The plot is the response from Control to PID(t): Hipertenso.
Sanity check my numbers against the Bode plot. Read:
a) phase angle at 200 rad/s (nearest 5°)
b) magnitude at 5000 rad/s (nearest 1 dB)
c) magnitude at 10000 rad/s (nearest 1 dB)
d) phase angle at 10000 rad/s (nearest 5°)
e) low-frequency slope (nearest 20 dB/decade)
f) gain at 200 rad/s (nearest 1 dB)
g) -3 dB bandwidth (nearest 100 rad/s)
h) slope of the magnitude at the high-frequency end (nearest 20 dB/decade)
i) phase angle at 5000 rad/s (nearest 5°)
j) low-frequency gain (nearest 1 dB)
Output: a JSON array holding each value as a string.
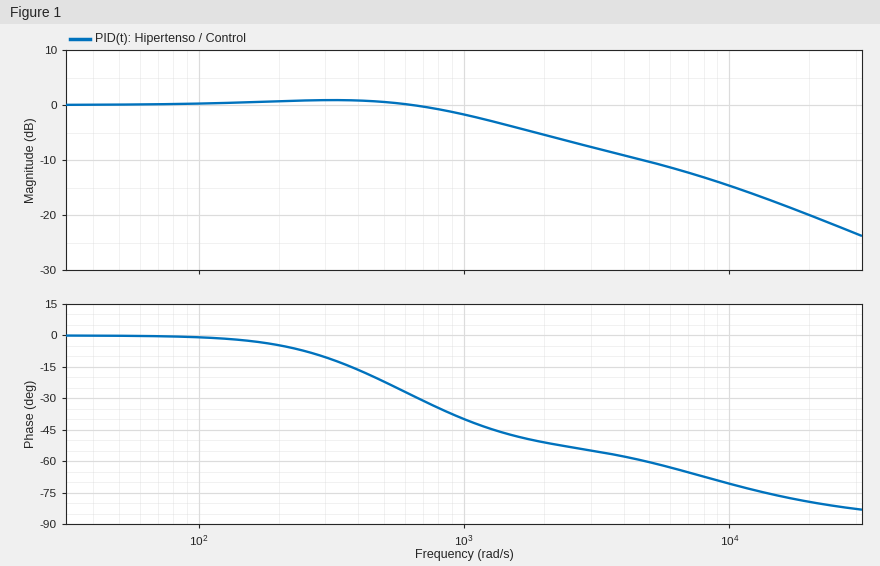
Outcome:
["-5°", "-10 dB", "-15 dB", "-70°", "0 dB/decade", "1 dB", "1300 rad/s", "-20 dB/decade", "-60°", "0 dB"]
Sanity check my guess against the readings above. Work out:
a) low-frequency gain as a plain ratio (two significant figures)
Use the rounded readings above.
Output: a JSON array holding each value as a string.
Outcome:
["1.0"]
